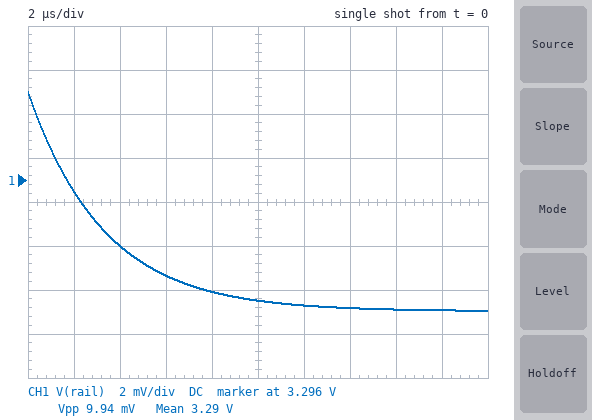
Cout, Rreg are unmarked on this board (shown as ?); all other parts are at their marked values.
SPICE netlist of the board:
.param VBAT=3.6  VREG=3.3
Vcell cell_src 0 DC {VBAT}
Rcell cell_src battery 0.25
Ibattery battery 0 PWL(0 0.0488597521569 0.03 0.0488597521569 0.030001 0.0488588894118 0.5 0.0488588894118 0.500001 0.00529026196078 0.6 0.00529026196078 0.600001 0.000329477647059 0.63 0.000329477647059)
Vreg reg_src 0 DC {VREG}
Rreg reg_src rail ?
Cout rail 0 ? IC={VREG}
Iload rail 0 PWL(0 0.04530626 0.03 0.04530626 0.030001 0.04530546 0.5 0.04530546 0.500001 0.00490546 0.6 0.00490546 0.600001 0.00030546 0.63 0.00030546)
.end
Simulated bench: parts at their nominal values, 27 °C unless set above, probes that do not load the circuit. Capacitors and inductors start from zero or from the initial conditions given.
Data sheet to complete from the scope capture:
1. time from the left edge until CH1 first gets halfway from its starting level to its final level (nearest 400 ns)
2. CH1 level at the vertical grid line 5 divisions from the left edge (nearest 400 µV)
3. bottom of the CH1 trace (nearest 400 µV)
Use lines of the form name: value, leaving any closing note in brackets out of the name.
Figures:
time from the left edge until CH1 first gets halfway from its starting level to its final level: 2.4 µs
CH1 level at the vertical grid line 5 divisions from the left edge: 3.2904 V
bottom of the CH1 trace: 3.2900 V
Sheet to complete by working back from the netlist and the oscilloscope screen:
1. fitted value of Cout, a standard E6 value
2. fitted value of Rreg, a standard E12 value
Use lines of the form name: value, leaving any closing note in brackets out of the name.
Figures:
fitted value of Cout, a standard E6 value: 15 µF
fitted value of Rreg, a standard E12 value: 0.22 Ω
